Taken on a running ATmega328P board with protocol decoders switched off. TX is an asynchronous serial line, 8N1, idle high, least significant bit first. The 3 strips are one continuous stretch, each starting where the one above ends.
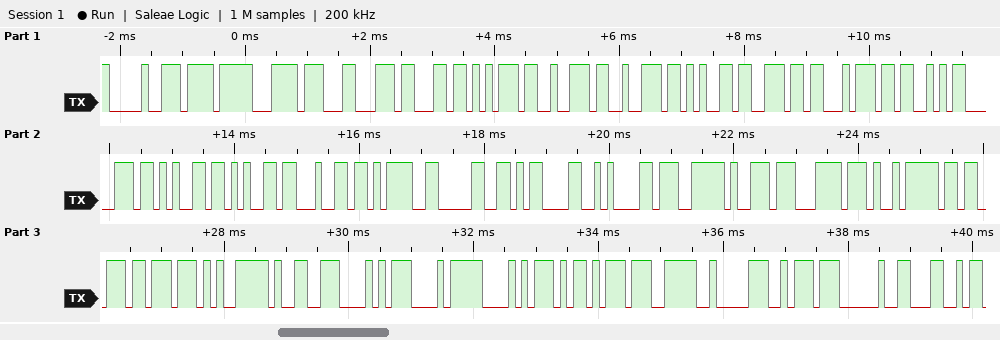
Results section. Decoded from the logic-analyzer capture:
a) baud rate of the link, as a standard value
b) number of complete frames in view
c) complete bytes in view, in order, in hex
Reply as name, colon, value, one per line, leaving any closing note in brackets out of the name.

baud rate of the link, as a standard value: 9600 baud
number of complete frames in view: 37
complete bytes in view, in order, in hex: 90 EF BC 8C 63 75 72 72 65 6E 74 53 70 65 65 64 3D 30 0D 0A E7 B9 BC E9 9B BB E5 99 A8 E8 A8 AD E7 82 BA 20 4C
